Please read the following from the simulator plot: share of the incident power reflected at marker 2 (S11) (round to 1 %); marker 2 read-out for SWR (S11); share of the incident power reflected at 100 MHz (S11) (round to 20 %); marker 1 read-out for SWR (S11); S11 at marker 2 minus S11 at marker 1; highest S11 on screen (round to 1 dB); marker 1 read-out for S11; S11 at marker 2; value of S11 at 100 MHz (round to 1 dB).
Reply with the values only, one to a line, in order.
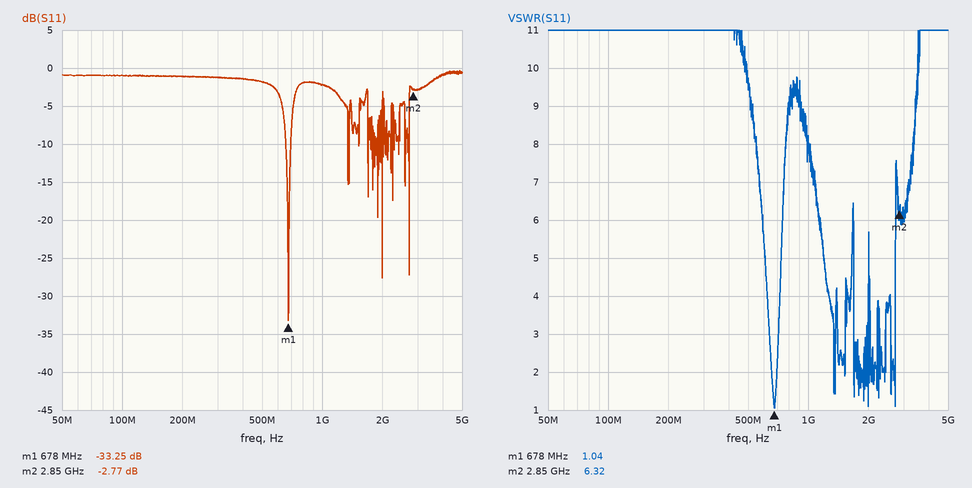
53 %
6.32
80 %
1.04
30.48 dB
0 dB
-33.25 dB
-2.77 dB
-1 dB
